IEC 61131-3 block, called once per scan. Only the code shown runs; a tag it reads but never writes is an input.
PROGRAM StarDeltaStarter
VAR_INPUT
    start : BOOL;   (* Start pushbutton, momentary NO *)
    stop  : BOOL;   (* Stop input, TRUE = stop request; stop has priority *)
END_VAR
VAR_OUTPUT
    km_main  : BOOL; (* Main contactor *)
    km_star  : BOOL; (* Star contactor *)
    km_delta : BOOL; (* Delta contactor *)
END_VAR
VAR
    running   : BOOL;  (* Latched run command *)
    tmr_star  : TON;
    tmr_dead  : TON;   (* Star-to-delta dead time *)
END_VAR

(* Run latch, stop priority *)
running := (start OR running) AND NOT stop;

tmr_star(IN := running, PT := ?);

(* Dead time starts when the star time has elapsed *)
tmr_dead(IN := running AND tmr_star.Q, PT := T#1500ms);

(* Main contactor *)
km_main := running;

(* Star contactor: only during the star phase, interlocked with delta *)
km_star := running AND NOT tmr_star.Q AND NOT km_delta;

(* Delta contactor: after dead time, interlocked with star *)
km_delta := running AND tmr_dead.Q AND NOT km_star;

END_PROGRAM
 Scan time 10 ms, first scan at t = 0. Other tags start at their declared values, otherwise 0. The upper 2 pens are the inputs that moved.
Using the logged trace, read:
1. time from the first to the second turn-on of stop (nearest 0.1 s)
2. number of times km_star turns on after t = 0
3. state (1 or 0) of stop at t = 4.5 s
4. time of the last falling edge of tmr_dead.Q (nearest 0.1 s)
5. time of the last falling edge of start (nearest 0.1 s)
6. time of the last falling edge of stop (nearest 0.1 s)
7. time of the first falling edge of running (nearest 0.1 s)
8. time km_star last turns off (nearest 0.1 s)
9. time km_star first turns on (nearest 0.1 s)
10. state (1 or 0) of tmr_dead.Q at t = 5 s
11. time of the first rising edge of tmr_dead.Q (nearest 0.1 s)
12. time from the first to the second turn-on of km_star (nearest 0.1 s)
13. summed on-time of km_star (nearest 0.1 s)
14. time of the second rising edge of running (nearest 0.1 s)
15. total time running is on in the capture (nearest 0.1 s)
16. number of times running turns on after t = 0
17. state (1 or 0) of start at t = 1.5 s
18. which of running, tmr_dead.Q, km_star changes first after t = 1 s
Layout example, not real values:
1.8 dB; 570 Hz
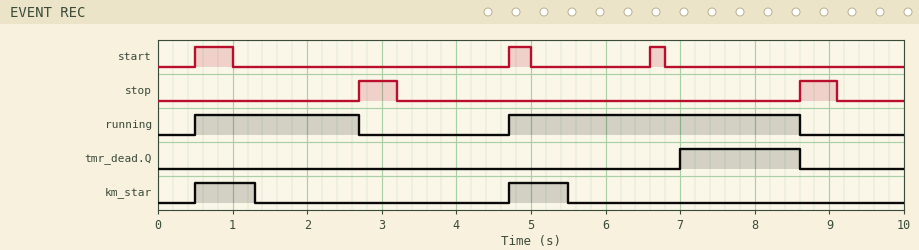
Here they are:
5.9 s; 2; 0; 8.6 s; 6.8 s; 9.1 s; 2.7 s; 5.5 s; 0.5 s; 0; 7.0 s; 4.2 s; 1.6 s; 4.7 s; 6.1 s; 2; 0; km_star
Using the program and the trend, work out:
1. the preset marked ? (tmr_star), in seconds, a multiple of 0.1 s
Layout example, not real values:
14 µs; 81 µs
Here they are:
0.8 s
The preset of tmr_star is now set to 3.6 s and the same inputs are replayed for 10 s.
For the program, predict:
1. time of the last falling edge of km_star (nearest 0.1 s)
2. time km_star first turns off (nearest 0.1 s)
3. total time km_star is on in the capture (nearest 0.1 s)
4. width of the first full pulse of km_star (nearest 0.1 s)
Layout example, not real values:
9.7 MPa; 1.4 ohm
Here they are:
8.3 s; 2.7 s; 5.8 s; 2.2 s
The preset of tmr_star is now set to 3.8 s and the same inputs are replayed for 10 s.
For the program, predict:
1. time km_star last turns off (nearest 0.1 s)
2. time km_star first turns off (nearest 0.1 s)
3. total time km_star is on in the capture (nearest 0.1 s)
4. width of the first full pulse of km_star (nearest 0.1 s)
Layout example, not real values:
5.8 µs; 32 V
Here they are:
8.5 s; 2.7 s; 6.0 s; 2.2 s
